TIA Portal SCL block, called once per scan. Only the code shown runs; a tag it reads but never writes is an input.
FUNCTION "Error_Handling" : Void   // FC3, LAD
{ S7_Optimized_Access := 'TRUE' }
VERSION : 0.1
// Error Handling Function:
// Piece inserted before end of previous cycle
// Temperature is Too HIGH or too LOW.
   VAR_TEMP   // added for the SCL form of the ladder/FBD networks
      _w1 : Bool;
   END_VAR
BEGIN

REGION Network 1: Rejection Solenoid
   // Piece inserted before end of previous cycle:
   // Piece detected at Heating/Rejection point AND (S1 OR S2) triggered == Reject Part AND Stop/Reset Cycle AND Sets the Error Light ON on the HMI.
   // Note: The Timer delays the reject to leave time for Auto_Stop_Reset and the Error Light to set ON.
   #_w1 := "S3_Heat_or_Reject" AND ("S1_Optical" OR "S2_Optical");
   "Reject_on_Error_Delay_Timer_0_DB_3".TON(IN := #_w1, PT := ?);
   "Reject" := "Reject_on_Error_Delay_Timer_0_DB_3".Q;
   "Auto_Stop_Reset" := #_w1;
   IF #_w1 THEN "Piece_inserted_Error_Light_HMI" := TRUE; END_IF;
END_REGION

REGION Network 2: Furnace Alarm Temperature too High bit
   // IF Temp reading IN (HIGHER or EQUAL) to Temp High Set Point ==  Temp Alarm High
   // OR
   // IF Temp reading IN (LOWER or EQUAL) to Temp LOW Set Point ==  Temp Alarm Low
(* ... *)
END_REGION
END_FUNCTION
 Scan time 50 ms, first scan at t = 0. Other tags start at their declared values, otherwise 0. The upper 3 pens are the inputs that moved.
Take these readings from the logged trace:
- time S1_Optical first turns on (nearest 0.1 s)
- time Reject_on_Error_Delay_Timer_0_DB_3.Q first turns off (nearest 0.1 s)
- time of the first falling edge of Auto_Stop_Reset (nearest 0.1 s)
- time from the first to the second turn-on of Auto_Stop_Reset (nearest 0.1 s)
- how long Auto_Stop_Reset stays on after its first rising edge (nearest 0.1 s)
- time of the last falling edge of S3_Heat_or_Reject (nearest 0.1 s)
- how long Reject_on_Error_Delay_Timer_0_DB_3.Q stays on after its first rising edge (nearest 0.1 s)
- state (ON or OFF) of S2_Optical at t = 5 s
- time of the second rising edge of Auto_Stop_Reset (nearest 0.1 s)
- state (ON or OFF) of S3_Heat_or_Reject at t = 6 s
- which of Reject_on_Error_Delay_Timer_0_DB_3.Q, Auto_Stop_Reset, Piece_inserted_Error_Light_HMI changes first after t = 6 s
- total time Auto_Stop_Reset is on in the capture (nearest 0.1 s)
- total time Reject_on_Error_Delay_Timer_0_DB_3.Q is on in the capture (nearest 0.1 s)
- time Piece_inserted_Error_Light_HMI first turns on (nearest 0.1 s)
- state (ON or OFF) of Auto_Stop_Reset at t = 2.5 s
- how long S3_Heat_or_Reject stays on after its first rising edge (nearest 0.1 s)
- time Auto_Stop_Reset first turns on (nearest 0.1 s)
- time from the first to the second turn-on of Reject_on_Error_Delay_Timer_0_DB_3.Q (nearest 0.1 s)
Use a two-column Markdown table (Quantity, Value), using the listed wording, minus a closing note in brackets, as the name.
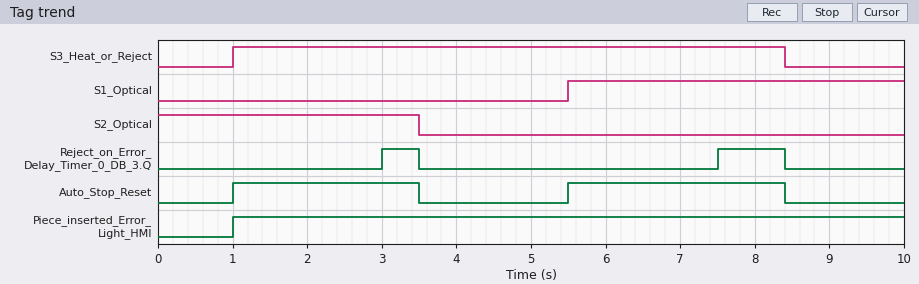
| Quantity | Value |
|---|---|
| time S1_Optical first turns on | 5.5 s |
| time Reject_on_Error_Delay_Timer_0_DB_3.Q first turns off | 3.5 s |
| time of the first falling edge of Auto_Stop_Reset | 3.5 s |
| time from the first to the second turn-on of Auto_Stop_Reset | 4.5 s |
| how long Auto_Stop_Reset stays on after its first rising edge | 2.5 s |
| time of the last falling edge of S3_Heat_or_Reject | 8.4 s |
| how long Reject_on_Error_Delay_Timer_0_DB_3.Q stays on after its first rising edge | 0.5 s |
| state (ON or OFF) of S2_Optical at t = 5 s | OFF |
| time of the second rising edge of Auto_Stop_Reset | 5.5 s |
| state (ON or OFF) of S3_Heat_or_Reject at t = 6 s | ON |
| which of Reject_on_Error_Delay_Timer_0_DB_3.Q, Auto_Stop_Reset, Piece_inserted_Error_Light_HMI changes first after t = 6 s | Reject_on_Error_Delay_Timer_0_DB_3.Q |
| total time Auto_Stop_Reset is on in the capture | 5.4 s |
| total time Reject_on_Error_Delay_Timer_0_DB_3.Q is on in the capture | 1.4 s |
| time Piece_inserted_Error_Light_HMI first turns on | 1.0 s |
| state (ON or OFF) of Auto_Stop_Reset at t = 2.5 s | ON |
| how long S3_Heat_or_Reject stays on after its first rising edge | 7.4 s |
| time Auto_Stop_Reset first turns on | 1.0 s |
| time from the first to the second turn-on of Reject_on_Error_Delay_Timer_0_DB_3.Q | 4.5 s |
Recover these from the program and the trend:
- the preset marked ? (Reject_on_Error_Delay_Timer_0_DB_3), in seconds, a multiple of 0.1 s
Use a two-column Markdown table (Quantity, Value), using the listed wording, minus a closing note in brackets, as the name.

| Quantity | Value |
|---|---|
| the preset marked ? (Reject_on_Error_Delay_Timer_0_DB_3), in seconds, a multiple of 0.1 s | 2.0 s |
